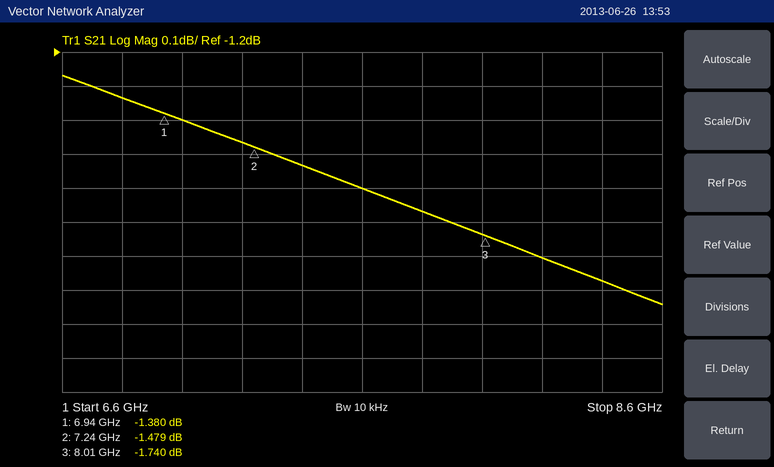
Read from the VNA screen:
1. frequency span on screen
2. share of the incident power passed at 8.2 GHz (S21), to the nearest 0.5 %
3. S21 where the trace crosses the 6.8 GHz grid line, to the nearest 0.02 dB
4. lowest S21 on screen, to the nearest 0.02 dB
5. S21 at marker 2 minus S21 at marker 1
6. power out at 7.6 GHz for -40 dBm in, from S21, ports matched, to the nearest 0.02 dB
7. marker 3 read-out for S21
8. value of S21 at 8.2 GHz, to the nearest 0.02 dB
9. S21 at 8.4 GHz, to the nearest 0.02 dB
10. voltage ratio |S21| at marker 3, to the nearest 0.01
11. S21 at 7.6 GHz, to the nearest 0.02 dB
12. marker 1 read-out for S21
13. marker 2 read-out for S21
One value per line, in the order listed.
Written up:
2 GHz
66.0 %
-1.34 dB
-1.94 dB
-0.099 dB
-41.60 dBm
-1.740 dB
-1.80 dB
-1.88 dB
0.82
-1.60 dB
-1.380 dB
-1.479 dB
